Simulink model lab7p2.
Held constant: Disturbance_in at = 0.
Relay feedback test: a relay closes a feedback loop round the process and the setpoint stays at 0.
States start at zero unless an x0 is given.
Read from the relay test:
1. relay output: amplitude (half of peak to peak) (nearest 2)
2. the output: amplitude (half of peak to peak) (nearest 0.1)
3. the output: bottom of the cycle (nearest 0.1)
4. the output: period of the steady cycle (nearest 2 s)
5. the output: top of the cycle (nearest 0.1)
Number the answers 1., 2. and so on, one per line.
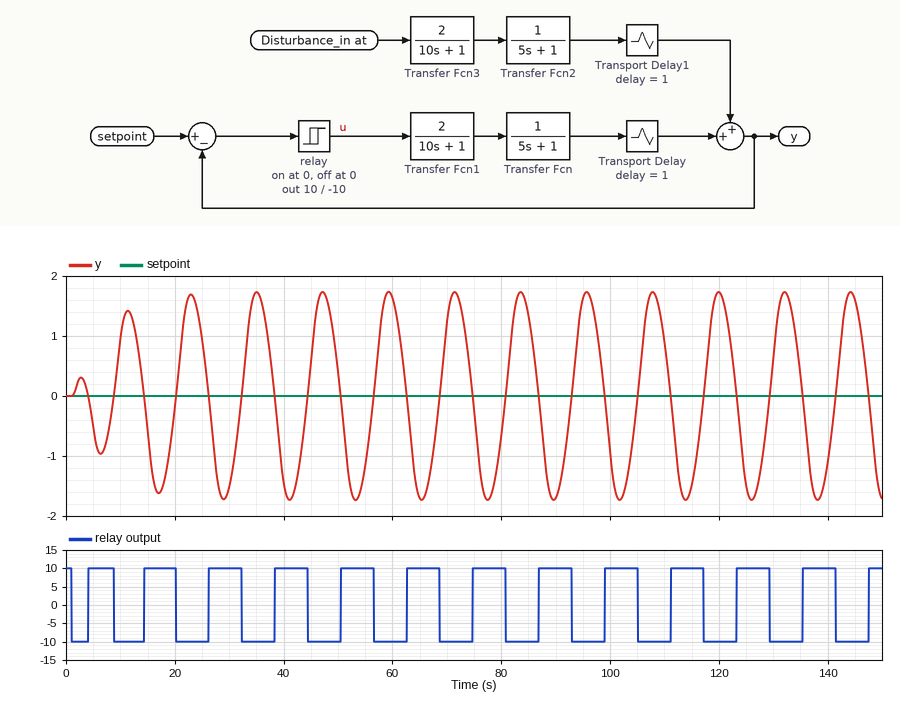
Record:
1. 10
2. 1.7
3. -1.7
4. 12 s
5. 1.7
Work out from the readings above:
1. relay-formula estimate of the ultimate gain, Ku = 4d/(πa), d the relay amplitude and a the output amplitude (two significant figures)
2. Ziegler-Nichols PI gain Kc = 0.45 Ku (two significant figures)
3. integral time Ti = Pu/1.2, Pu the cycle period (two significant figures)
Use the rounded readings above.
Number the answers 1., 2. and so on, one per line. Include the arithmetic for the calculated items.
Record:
1. 4 × 10 / (π × 1.7) = 7.5
2. 0.45 × 7.5 = 3.4
3. 12 / 1.2 = 10 s
